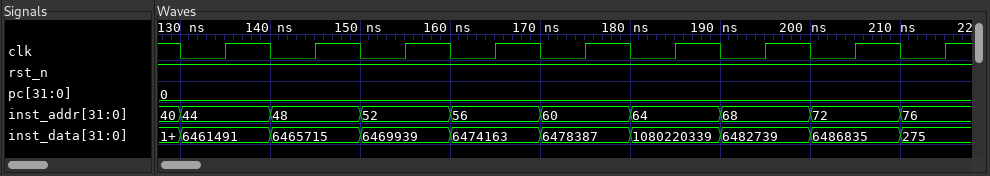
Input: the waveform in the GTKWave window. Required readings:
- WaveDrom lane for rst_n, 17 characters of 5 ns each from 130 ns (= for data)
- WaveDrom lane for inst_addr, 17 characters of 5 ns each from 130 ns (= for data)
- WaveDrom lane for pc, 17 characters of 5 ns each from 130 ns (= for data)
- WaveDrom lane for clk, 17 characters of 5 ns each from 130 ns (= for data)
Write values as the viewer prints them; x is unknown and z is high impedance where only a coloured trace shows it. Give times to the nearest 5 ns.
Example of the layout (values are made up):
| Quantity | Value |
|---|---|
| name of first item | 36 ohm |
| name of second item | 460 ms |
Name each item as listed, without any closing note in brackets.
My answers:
| Quantity | Value |
|---|---|
| WaveDrom lane for rst_n, 17 characters of 5 ns each from 130 ns | {name: 'rst_n', wave: '1................'} |
| WaveDrom lane for inst_addr, 17 characters of 5 ns each from 130 ns | {name: 'inst_addr', wave: '=.=.=.=.=.=.=.=.=', data: '44 48 52 56 60 64 68 72 76'} |
| WaveDrom lane for pc, 17 characters of 5 ns each from 130 ns | {name: 'pc', wave: '=................', data: '0'} |
| WaveDrom lane for clk, 17 characters of 5 ns each from 130 ns | {name: 'clk', wave: '01010101010101010'} |
